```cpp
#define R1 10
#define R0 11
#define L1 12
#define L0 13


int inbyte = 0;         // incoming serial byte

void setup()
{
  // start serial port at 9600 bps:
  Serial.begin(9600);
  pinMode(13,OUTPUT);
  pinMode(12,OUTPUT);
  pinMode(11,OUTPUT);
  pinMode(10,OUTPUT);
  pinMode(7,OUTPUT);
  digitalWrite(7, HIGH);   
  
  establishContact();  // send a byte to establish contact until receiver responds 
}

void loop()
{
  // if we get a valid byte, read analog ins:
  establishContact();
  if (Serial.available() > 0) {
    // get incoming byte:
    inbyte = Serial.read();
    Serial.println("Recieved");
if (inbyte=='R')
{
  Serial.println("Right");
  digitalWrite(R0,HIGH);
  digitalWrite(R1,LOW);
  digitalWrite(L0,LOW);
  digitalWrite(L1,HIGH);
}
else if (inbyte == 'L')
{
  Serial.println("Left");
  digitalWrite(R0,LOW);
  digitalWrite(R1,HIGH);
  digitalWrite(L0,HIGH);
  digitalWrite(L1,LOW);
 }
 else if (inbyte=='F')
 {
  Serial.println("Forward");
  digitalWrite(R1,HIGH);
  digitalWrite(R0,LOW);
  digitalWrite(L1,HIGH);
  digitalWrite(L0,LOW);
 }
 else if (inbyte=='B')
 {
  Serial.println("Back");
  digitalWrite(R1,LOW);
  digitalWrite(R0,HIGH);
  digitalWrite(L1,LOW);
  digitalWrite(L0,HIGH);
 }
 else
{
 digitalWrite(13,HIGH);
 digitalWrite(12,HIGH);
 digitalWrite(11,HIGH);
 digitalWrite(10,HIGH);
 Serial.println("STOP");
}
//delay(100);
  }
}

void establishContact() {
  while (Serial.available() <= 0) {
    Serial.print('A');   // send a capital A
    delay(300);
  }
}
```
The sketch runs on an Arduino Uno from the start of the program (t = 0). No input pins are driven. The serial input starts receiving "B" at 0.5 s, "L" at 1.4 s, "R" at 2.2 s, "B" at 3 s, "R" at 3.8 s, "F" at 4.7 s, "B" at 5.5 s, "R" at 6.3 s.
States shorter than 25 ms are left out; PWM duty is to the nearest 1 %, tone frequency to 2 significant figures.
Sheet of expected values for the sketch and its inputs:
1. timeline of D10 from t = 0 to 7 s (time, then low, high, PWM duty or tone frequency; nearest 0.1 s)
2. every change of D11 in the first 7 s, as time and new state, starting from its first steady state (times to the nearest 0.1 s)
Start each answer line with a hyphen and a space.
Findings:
- 0 s low; 1.5 s high; 2.4 s low; 4.8 s high; 5.7 s low
- 0 s low; 0.6 s high; 1.5 s low; 2.4 s high; 4.8 s low; 5.7 s high
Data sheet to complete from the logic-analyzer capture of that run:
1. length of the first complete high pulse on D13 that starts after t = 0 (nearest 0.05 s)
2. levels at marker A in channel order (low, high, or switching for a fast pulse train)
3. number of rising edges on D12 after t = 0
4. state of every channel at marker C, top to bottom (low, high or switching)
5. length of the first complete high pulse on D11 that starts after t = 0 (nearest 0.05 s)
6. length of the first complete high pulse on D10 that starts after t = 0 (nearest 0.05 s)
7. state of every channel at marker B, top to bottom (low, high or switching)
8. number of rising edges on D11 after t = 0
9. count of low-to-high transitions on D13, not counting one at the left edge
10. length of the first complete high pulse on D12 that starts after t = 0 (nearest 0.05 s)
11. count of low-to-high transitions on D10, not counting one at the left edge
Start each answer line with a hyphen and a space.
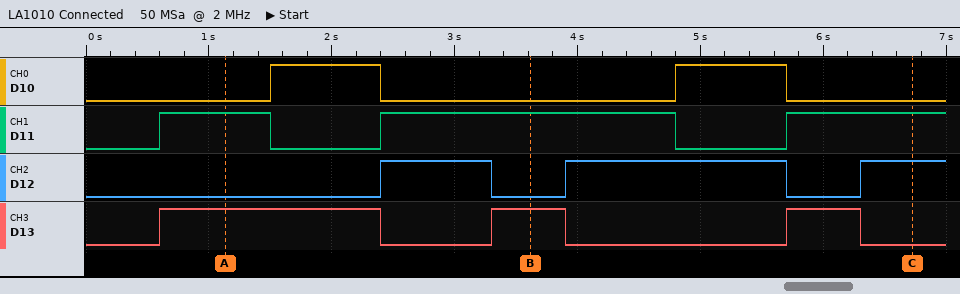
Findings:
- 1.80 s
- D10 low, D11 high, D12 low, D13 high
- 3
- D10 low, D11 high, D12 high, D13 low
- 0.90 s
- 0.90 s
- D10 low, D11 high, D12 low, D13 high
- 3
- 3
- 0.90 s
- 2
